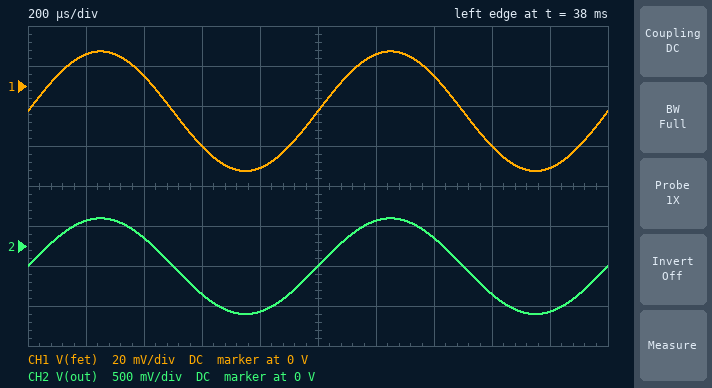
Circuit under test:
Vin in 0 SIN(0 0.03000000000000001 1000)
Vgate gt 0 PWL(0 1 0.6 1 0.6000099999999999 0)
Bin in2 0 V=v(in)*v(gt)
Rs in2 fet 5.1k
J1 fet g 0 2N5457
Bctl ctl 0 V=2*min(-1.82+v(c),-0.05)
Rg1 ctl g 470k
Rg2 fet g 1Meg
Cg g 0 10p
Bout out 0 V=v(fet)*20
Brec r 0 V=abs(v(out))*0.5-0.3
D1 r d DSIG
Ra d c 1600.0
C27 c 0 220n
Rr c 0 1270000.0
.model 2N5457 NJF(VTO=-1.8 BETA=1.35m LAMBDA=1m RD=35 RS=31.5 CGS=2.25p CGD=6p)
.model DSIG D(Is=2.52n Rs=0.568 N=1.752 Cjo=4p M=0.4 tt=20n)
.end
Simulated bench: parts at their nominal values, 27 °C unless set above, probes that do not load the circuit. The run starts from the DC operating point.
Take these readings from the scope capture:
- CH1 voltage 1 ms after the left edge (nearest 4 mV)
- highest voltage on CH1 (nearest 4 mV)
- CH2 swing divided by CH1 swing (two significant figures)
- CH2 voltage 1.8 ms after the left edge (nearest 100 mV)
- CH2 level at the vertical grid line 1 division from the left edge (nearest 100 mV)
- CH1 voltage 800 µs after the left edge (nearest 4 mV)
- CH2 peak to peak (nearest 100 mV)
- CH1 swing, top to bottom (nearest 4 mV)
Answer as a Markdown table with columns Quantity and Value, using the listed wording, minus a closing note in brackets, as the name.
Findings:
| Quantity | Value |
|---|---|
| CH1 voltage 1 ms after the left edge | -12 mV |
| highest voltage on CH1 | 16 mV |
| CH2 swing divided by CH1 swing | 20 |
| CH2 voltage 1.8 ms after the left edge | -800 mV |
| CH2 level at the vertical grid line 1 division from the left edge | 300 mV |
| CH1 voltage 800 µs after the left edge | -40 mV |
| CH2 peak to peak | 1.2 V |
| CH1 swing, top to bottom | 60 mV |
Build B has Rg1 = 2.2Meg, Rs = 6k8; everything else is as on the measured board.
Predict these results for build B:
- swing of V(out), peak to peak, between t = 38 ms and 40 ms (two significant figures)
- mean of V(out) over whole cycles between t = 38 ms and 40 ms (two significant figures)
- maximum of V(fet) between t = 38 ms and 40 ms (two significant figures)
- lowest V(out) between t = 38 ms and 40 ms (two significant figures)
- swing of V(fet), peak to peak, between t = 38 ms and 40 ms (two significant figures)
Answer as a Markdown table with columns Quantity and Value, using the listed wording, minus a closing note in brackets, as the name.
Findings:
| Quantity | Value |
|---|---|
| swing of V(out), peak to peak, between t = 38 ms and 40 ms | 100 mV |
| mean of V(out) over whole cycles between t = 38 ms and 40 ms | -13 mV |
| maximum of V(fet) between t = 38 ms and 40 ms | 1.9 mV |
| lowest V(out) between t = 38 ms and 40 ms | -64 mV |
| swing of V(fet), peak to peak, between t = 38 ms and 40 ms | 5.1 mV |
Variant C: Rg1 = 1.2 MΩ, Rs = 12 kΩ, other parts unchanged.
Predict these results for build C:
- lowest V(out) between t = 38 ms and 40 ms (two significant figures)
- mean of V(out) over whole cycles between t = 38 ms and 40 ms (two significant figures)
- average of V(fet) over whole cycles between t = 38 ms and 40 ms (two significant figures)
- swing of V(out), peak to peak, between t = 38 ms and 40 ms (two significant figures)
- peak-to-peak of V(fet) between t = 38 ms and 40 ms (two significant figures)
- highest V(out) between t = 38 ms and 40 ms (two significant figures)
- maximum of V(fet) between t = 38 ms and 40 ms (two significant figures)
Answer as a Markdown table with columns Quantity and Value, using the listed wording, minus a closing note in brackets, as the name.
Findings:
| Quantity | Value |
|---|---|
| lowest V(out) between t = 38 ms and 40 ms | -180 mV |
| mean of V(out) over whole cycles between t = 38 ms and 40 ms | -72 mV |
| average of V(fet) over whole cycles between t = 38 ms and 40 ms | -3.6 mV |
| swing of V(out), peak to peak, between t = 38 ms and 40 ms | 220 mV |
| peak-to-peak of V(fet) between t = 38 ms and 40 ms | 11 mV |
| highest V(out) between t = 38 ms and 40 ms | 37 mV |
| maximum of V(fet) between t = 38 ms and 40 ms | 1.8 mV |
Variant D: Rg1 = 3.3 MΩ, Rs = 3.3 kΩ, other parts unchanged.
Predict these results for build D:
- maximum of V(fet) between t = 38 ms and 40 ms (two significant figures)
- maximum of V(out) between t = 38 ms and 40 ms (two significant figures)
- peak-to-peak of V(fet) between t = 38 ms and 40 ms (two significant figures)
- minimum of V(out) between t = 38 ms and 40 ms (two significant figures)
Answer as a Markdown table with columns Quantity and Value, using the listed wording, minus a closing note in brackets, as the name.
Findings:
| Quantity | Value |
|---|---|
| maximum of V(fet) between t = 38 ms and 40 ms | 3.3 mV |
| maximum of V(out) between t = 38 ms and 40 ms | 66 mV |
| peak-to-peak of V(fet) between t = 38 ms and 40 ms | 7.3 mV |
| minimum of V(out) between t = 38 ms and 40 ms | -80 mV |
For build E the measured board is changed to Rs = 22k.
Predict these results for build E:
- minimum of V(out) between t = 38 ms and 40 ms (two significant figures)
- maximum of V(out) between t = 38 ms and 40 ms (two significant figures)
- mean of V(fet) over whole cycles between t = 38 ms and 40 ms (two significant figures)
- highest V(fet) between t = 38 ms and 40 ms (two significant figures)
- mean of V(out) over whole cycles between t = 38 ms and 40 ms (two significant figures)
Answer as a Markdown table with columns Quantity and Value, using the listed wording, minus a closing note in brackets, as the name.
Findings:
| Quantity | Value |
|---|---|
| minimum of V(out) between t = 38 ms and 40 ms | -1.6 V |
| maximum of V(out) between t = 38 ms and 40 ms | -380 mV |
| mean of V(fet) over whole cycles between t = 38 ms and 40 ms | -48 mV |
| highest V(fet) between t = 38 ms and 40 ms | -19 mV |
| mean of V(out) over whole cycles between t = 38 ms and 40 ms | -970 mV |
